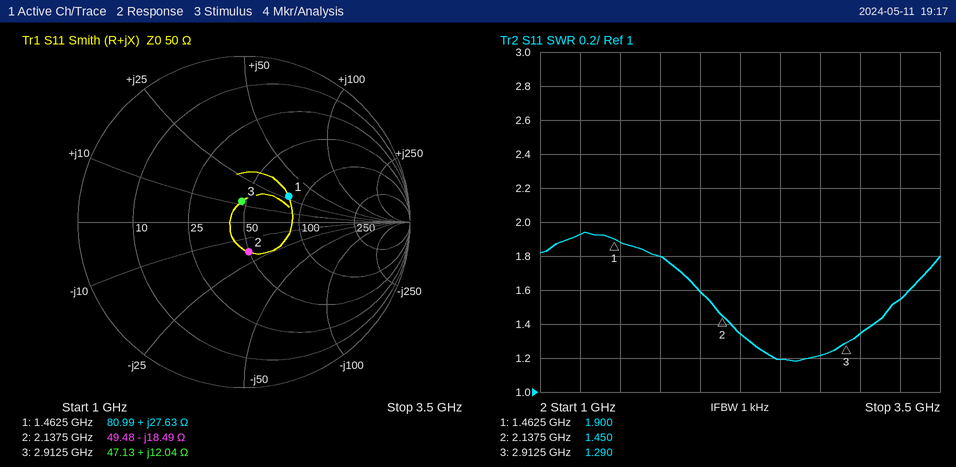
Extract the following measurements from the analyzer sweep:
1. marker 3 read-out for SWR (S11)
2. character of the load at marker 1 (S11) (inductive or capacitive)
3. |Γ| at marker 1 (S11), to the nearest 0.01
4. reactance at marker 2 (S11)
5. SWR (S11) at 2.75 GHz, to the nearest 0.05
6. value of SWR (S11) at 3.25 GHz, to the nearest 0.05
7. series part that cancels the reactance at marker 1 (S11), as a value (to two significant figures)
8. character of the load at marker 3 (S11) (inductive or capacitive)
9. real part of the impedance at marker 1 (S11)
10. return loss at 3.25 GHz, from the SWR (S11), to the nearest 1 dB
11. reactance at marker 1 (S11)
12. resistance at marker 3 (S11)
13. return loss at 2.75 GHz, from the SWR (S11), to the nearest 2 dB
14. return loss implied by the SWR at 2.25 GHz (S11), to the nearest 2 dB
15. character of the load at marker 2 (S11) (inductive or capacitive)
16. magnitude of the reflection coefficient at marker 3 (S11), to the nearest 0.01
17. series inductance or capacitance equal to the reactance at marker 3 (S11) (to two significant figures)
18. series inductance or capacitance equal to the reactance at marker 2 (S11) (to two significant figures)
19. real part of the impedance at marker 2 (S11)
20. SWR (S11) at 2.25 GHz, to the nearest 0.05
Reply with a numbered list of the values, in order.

1. 1.290
2. inductive
3. 0.31
4. -18.49 Ω
5. 1.20
6. 1.55
7. 3.9 pF
8. inductive
9. 80.99 Ω
10. 13 dB
11. +27.63 Ω
12. 47.13 Ω
13. 20 dB
14. 16 dB
15. capacitive
16. 0.13
17. 660 pH
18. 4.0 pF
19. 49.48 Ω
20. 1.35
